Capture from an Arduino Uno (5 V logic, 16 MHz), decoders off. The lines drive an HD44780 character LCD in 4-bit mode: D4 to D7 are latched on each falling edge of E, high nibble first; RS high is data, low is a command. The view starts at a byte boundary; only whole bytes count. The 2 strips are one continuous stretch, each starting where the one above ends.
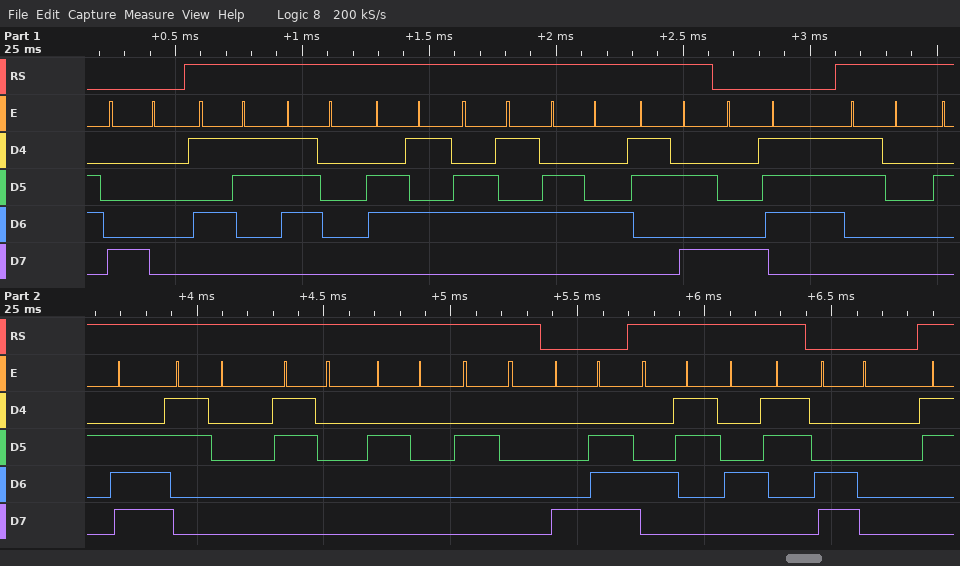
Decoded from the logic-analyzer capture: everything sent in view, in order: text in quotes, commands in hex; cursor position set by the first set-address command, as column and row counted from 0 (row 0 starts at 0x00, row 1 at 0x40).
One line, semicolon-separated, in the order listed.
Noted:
0x80 "Speed:" 0x87 "0.00  " 0x8E "CC" 0xC0; column 0, row 0
